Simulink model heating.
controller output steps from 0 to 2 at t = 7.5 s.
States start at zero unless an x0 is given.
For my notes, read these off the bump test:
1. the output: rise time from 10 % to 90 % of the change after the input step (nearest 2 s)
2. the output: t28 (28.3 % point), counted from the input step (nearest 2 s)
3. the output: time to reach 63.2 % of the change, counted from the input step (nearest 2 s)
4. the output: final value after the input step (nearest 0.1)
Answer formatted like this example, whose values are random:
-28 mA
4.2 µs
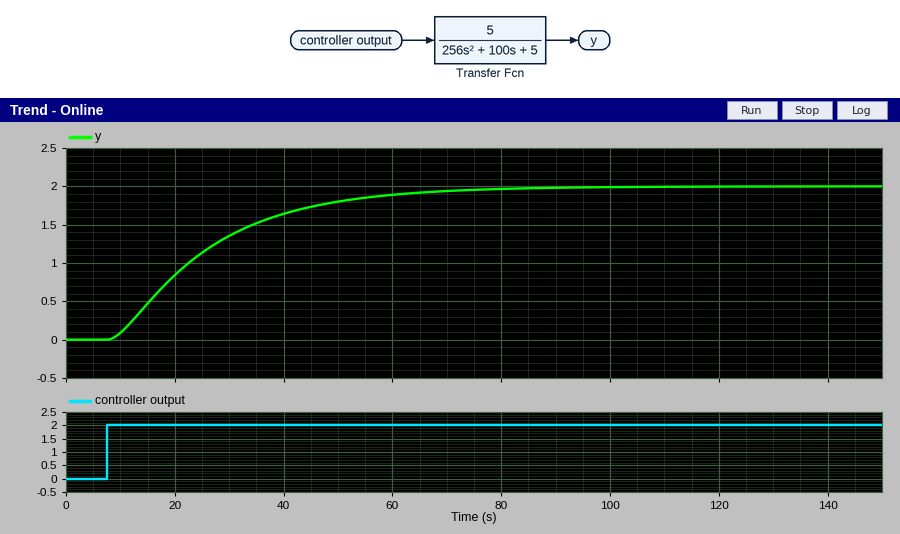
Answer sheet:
38 s
8 s
20 s
2.0
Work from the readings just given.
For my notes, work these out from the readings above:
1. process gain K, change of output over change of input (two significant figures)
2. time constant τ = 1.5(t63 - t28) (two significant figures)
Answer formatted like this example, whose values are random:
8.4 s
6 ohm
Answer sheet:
1.0
18 s
